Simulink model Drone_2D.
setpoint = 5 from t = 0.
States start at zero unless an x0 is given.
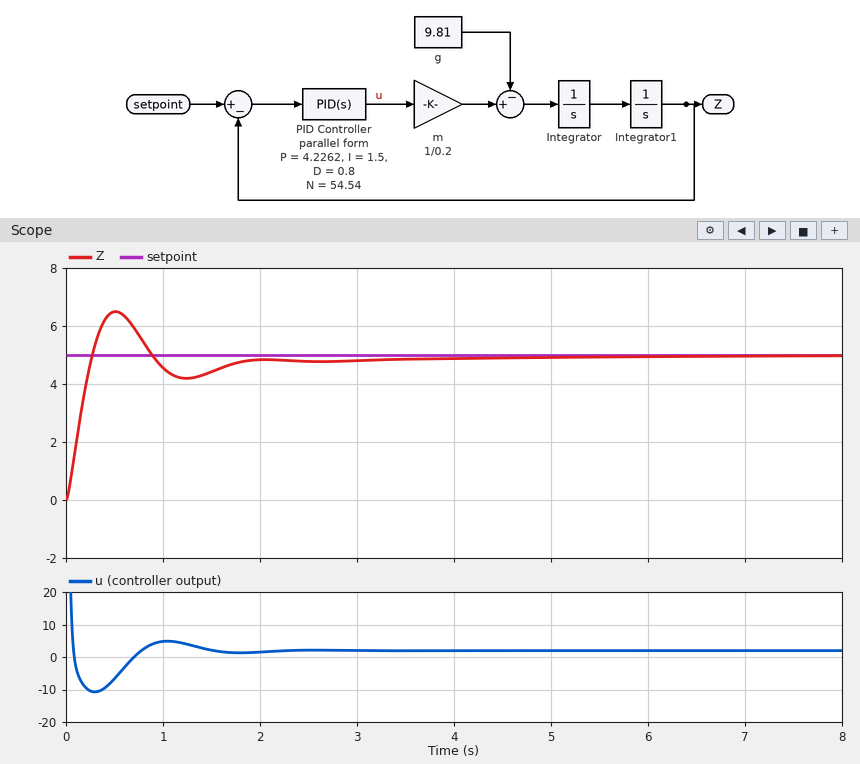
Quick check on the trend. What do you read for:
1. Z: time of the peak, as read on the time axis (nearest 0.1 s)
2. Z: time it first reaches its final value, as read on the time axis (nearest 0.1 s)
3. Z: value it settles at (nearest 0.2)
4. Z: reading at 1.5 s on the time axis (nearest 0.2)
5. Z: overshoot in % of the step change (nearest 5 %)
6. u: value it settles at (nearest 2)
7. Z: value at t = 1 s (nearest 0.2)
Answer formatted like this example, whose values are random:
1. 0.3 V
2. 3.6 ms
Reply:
1. 0.5 s
2. 0.3 s
3. 5.0
4. 4.4
5. 30 %
6. 2
7. 4.6
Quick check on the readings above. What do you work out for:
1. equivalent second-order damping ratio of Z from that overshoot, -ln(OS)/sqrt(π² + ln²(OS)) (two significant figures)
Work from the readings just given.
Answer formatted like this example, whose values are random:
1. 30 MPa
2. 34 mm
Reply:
1. 0.36
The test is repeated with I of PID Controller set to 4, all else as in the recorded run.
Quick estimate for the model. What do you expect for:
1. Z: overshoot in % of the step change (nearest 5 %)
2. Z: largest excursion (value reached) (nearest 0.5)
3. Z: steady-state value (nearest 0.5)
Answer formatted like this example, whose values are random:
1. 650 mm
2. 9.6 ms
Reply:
1. 35 %
2. 7.0
3. 5.0
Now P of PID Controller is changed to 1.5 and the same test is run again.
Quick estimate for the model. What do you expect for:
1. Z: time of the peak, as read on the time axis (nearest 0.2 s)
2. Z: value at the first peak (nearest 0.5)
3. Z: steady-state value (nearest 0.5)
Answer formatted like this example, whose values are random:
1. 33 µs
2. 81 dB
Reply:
1. 0.8 s
2. 5.5
3. 5.0
